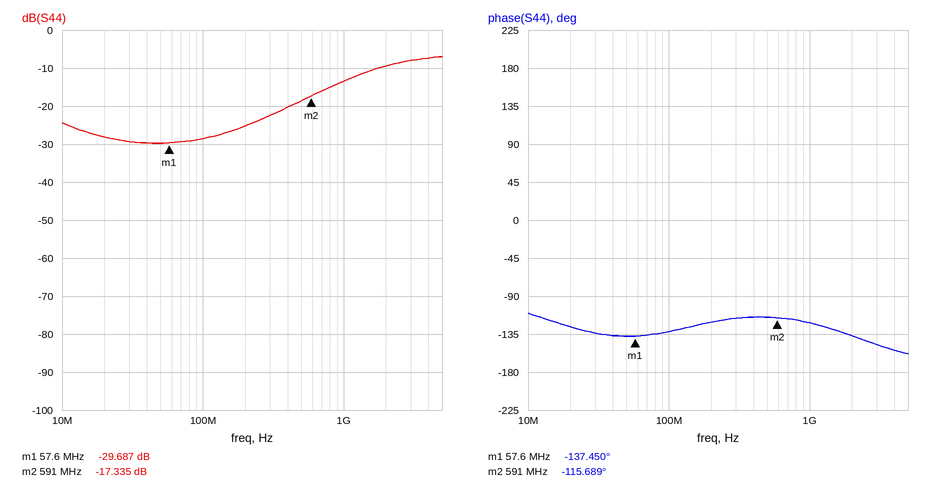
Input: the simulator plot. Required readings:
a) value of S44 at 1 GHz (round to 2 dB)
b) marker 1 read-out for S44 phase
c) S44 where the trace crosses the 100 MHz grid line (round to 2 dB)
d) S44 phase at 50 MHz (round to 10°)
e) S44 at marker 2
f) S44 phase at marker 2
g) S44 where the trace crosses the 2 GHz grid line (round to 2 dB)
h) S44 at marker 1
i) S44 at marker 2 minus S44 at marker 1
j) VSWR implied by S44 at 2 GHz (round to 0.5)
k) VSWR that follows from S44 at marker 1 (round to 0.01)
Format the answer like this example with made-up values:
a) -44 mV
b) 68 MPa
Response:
a) -14 dB
b) -137.450°
c) -28 dB
d) -140°
e) -17.335 dB
f) -115.689°
g) -10 dB
h) -29.687 dB
i) 12.352 dB
j) 2.0
k) 1.07
